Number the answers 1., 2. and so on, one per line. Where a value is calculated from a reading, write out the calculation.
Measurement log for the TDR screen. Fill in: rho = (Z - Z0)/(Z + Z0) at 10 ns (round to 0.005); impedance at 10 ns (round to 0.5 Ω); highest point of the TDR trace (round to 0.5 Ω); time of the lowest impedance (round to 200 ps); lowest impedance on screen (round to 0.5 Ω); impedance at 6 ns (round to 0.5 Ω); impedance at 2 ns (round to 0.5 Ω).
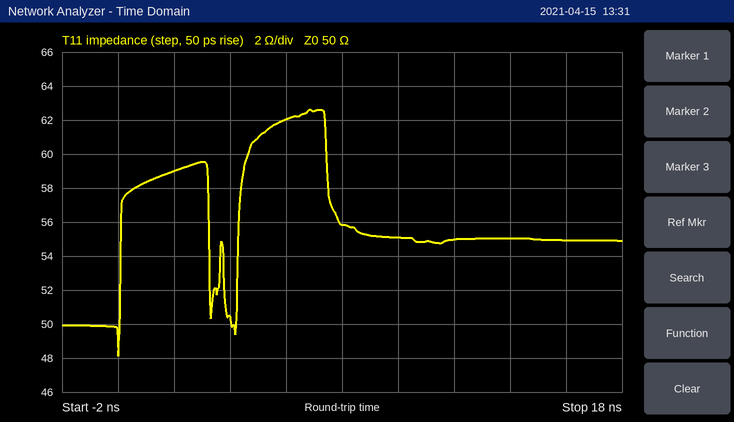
1. (55 − 50)/(55 + 50) ≈ +0.0476, so +0.050 to the nearest 0.005
2. 55.0 Ω
3. 62.5 Ω
4. 0.0 ns
5. 48.0 Ω
6. 62.0 Ω
7. 59.0 Ω
